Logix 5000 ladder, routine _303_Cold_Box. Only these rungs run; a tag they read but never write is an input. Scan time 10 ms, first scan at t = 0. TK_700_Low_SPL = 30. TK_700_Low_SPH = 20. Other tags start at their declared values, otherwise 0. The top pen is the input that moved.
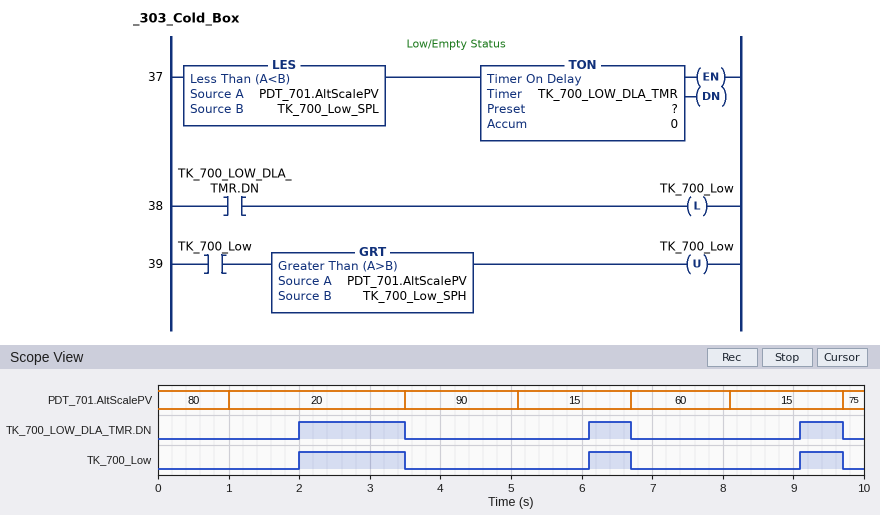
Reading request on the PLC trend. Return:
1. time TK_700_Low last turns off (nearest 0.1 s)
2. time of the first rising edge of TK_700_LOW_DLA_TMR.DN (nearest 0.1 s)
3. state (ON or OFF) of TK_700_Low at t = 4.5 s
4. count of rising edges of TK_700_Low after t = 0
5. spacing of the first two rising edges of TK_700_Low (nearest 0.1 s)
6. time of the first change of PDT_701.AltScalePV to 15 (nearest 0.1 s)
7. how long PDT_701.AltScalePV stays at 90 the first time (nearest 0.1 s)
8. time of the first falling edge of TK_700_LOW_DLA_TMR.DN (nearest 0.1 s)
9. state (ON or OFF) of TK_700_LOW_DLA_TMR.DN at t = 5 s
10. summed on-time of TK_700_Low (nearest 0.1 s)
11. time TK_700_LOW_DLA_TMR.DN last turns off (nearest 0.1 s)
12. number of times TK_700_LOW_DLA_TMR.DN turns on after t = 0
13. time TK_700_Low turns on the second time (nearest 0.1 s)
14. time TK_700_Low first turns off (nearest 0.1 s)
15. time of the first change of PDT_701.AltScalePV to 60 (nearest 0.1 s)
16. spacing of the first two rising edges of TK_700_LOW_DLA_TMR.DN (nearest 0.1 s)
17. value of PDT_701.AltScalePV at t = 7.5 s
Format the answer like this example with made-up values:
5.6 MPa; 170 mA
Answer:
9.7 s; 2.0 s; OFF; 3; 4.1 s; 5.1 s; 1.6 s; 3.5 s; OFF; 2.7 s; 9.7 s; 3; 6.1 s; 3.5 s; 6.7 s; 4.1 s; 60
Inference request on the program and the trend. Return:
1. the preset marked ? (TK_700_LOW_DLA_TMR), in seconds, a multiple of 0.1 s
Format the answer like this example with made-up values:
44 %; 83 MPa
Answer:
1.0 s
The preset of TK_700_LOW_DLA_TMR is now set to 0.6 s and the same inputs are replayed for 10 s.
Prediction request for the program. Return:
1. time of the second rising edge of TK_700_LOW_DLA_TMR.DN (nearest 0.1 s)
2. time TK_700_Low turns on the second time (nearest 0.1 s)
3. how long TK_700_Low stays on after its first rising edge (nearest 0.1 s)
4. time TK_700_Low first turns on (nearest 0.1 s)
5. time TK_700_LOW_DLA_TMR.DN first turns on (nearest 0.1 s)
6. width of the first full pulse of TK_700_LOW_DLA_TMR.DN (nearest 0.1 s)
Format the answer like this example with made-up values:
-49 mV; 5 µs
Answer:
5.7 s; 5.7 s; 1.9 s; 1.6 s; 1.6 s; 1.9 s
